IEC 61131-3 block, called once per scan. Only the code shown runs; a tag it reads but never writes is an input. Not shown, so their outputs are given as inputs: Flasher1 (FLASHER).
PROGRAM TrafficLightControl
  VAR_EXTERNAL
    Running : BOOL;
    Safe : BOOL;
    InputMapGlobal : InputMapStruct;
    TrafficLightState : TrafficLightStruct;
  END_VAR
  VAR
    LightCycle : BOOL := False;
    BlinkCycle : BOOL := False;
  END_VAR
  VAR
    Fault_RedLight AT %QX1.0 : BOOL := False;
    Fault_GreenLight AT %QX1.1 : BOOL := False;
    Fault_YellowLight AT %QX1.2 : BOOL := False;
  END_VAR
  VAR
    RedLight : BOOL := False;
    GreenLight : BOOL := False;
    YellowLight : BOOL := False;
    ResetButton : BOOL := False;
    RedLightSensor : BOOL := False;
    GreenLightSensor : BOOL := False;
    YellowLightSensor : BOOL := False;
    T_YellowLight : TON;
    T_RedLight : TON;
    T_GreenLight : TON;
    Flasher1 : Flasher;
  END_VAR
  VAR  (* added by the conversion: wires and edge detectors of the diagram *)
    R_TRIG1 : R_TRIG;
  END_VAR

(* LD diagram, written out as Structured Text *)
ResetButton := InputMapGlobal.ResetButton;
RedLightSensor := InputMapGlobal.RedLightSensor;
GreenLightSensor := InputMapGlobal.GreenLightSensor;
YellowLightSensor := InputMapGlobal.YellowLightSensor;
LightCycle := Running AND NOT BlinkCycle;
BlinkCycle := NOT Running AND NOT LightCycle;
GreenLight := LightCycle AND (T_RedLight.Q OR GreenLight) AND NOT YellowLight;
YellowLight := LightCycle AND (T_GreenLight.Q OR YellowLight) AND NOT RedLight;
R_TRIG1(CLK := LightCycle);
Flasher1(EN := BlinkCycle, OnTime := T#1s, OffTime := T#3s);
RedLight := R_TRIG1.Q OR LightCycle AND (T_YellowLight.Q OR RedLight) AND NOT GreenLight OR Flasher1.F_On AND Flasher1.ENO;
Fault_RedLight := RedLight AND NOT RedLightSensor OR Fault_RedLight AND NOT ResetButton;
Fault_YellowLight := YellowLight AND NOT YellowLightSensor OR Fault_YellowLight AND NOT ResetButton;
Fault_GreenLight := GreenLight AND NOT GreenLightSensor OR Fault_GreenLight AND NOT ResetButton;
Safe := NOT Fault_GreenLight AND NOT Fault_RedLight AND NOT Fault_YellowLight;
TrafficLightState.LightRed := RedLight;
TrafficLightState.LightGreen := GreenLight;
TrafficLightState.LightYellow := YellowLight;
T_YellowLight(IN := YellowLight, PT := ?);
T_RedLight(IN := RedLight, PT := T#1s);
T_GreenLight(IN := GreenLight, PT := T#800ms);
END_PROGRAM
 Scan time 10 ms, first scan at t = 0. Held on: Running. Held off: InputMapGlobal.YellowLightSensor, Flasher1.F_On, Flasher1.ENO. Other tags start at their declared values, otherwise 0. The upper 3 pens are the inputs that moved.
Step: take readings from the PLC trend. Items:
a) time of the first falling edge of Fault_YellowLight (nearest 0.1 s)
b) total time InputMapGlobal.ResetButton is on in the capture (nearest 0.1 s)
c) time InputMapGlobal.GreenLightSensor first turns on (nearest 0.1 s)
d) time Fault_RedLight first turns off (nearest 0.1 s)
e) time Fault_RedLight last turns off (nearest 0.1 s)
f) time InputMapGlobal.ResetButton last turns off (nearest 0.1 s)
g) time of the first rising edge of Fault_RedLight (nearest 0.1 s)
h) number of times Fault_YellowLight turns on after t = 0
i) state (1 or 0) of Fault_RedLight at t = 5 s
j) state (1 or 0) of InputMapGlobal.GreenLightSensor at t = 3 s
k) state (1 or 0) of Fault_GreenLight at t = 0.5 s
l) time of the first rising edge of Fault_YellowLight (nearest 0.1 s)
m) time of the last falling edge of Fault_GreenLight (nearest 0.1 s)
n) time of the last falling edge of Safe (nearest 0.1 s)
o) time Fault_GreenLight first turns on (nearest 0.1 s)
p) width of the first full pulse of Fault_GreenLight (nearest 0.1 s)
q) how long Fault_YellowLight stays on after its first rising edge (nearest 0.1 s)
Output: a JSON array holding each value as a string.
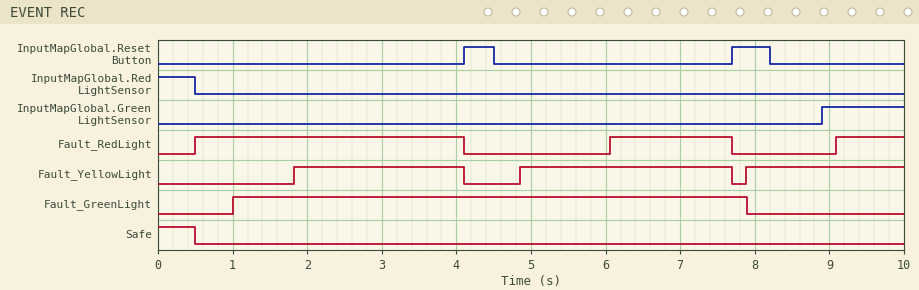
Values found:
["4.1 s", "0.9 s", "8.9 s", "4.1 s", "7.7 s", "8.2 s", "0.5 s", "3", "0", "0", "0", "1.8 s", "7.9 s", "0.5 s", "1.0 s", "6.9 s", "2.3 s"]
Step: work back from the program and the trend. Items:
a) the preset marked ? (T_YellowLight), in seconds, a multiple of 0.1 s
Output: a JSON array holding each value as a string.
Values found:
["1.2 s"]
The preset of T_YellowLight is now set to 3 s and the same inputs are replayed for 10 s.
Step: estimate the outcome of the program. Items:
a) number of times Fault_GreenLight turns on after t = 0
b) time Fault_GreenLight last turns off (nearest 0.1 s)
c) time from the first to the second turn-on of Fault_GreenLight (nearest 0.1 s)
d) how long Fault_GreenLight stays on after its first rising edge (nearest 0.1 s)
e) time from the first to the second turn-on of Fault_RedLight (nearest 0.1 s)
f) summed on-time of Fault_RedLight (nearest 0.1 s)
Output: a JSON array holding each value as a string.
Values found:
["2", "7.7 s", "4.8 s", "3.1 s", "4.3 s", "6.8 s"]
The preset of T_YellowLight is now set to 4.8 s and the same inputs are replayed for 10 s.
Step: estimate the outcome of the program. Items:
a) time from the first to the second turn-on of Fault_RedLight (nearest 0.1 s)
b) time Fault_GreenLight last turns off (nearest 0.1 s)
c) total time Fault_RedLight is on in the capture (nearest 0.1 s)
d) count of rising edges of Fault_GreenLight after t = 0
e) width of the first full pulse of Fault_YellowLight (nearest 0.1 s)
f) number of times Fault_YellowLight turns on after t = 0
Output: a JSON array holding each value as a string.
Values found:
["6.1 s", "4.1 s", "4.7 s", "2", "5.9 s", "2"]
